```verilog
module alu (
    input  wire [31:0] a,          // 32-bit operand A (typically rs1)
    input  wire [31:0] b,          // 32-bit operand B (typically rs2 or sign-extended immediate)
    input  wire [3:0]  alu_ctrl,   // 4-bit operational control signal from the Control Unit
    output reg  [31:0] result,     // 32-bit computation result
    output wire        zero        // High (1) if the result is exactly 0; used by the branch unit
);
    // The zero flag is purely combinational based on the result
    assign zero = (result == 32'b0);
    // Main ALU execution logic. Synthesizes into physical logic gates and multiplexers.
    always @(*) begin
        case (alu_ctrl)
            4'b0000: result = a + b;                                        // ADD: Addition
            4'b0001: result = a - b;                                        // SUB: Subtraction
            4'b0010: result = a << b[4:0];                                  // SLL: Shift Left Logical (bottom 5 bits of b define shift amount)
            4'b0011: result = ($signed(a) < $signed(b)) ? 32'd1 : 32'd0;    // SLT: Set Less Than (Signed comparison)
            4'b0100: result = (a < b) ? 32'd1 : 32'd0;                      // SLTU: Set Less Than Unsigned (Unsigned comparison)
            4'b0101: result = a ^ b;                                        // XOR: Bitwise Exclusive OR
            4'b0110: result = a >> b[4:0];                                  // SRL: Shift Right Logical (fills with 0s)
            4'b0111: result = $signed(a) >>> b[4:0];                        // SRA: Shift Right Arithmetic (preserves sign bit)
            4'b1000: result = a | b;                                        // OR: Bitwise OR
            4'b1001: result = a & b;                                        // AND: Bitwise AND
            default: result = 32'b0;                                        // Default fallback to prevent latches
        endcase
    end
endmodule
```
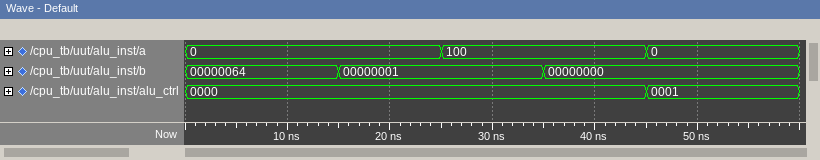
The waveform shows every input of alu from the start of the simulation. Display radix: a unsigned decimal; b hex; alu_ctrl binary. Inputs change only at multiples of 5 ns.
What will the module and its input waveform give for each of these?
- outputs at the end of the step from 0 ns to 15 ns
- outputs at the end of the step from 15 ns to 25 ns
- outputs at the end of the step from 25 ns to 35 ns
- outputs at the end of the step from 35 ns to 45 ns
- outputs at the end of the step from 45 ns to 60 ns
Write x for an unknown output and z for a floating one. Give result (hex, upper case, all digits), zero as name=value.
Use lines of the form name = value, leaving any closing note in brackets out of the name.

outputs at the end of the step from 0 ns to 15 ns = result=00000064, zero=0
outputs at the end of the step from 15 ns to 25 ns = result=00000001, zero=0
outputs at the end of the step from 25 ns to 35 ns = result=00000065, zero=0
outputs at the end of the step from 35 ns to 45 ns = result=00000064, zero=0
outputs at the end of the step from 45 ns to 60 ns = result=00000000, zero=1
